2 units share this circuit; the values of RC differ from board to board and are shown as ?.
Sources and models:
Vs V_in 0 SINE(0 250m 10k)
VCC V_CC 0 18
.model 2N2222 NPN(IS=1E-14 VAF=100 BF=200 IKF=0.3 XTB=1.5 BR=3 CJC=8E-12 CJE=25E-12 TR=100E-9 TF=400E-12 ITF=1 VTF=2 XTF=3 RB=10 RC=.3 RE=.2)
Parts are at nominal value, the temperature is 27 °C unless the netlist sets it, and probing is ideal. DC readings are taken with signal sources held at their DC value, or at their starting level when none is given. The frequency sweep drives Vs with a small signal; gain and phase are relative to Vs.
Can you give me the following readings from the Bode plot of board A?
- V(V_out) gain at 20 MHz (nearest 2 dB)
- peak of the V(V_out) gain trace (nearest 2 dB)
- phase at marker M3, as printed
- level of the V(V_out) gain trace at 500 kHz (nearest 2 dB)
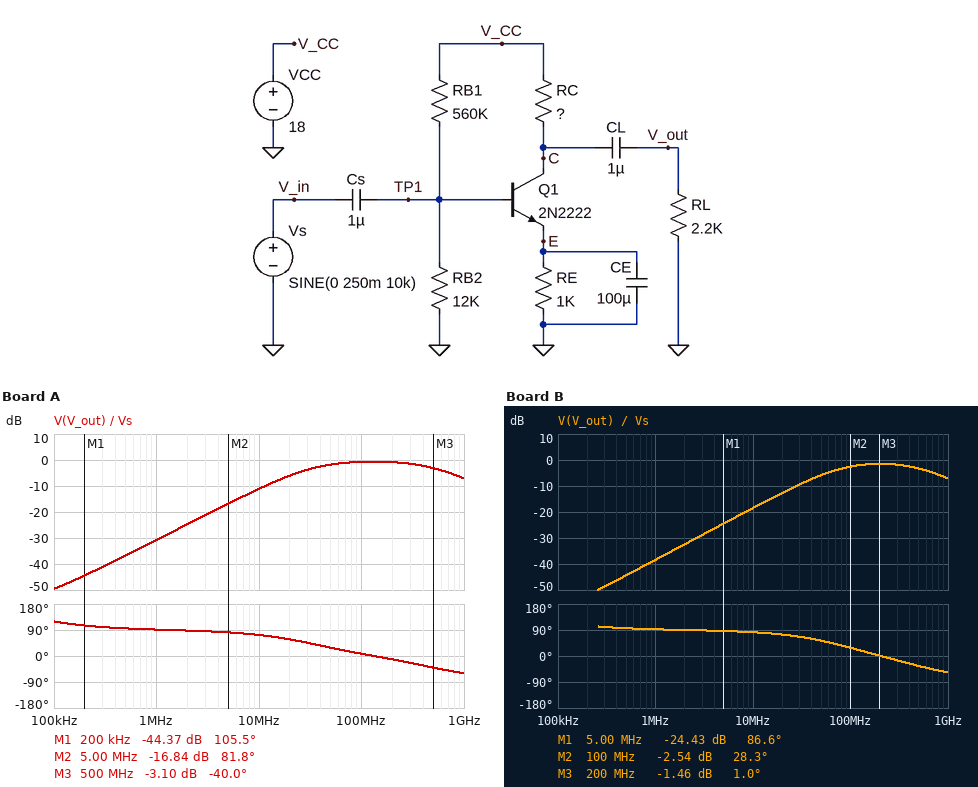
-6 dB
0 dB
-40.0 deg
-36 dB
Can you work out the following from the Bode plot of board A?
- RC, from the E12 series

6.8 kΩ
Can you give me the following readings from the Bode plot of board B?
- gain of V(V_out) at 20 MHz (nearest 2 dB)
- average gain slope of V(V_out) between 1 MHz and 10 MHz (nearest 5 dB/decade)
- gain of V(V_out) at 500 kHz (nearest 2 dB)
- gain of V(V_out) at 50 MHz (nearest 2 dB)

-12 dB
20 dB/decade
-44 dB
-6 dB
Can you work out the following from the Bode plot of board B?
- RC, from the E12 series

1 kΩ
